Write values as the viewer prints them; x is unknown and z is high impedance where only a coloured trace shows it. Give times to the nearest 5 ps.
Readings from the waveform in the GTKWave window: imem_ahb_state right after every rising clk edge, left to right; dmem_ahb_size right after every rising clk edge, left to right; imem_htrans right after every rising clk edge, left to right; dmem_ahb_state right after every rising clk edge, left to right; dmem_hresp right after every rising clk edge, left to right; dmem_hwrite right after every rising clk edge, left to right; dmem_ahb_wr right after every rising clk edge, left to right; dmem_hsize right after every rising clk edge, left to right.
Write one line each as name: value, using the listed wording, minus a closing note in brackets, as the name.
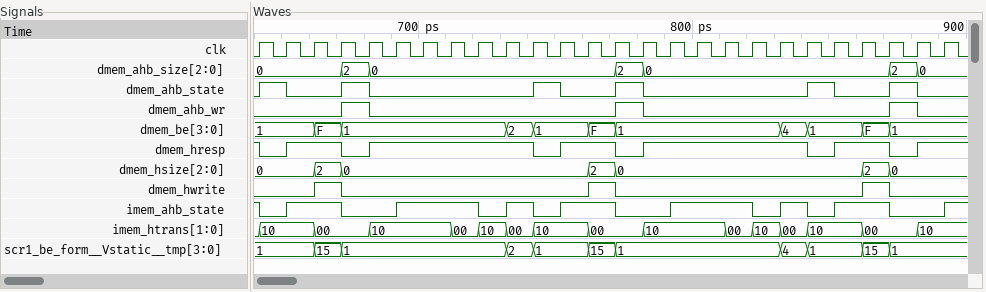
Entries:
imem_ahb_state right after every rising clk edge, left to right: 0 1 1 0 0 1 1 1 0 1 0 1 1 0 0 1 1 1 0 1 0 1 1 0 0 1
dmem_ahb_size right after every rising clk edge, left to right: 0, 0, 0, 2, 0, 0, 0, 0, 0, 0, 0, 0, 0, 2, 0, 0, 0, 0, 0, 0, 0, 0, 0, 2, 0, 0
imem_htrans right after every rising clk edge, left to right: 10, 10, 00, 00, 10, 10, 10, 00, 10, 00, 10, 10, 00, 00, 10, 10, 10, 00, 10, 00, 10, 10, 00, 00, 10, 10
dmem_ahb_state right after every rising clk edge, left to right: 1 0 0 1 0 0 0 0 0 0 1 0 0 1 0 0 0 0 0 0 1 0 0 1 0 0
dmem_hresp right after every rising clk edge, left to right: 0 1 1 0 1 1 1 1 1 1 0 1 1 0 1 1 1 1 1 1 0 1 1 0 1 1
dmem_hwrite right after every rising clk edge, left to right: 0 0 1 0 0 0 0 0 0 0 0 0 1 0 0 0 0 0 0 0 0 0 1 0 0 0
dmem_ahb_wr right after every rising clk edge, left to right: 0 0 0 1 0 0 0 0 0 0 0 0 0 1 0 0 0 0 0 0 0 0 0 1 0 0
dmem_hsize right after every rising clk edge, left to right: 0, 0, 2, 0, 0, 0, 0, 0, 0, 0, 0, 0, 2, 0, 0, 0, 0, 0, 0, 0, 0, 0, 2, 0, 0, 0
